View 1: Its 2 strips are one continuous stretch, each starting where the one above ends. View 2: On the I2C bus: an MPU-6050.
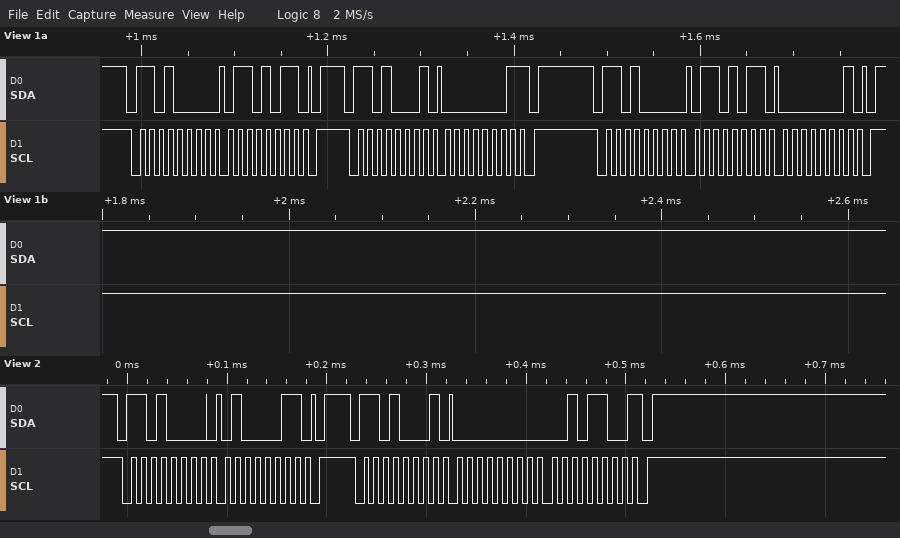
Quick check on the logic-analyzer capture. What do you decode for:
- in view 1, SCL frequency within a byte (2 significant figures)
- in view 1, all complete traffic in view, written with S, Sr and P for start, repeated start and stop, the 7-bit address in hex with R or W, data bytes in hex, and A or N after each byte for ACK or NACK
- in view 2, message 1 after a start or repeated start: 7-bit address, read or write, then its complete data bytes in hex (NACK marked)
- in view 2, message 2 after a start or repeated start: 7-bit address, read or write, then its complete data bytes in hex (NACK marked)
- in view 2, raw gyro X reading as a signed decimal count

100 kHz
S 68W A 6B A P S 68R A 01 N P S 68W A 6B A 01 A P
0x68 write: 43
0x68 read: 00 2C NACK
44
